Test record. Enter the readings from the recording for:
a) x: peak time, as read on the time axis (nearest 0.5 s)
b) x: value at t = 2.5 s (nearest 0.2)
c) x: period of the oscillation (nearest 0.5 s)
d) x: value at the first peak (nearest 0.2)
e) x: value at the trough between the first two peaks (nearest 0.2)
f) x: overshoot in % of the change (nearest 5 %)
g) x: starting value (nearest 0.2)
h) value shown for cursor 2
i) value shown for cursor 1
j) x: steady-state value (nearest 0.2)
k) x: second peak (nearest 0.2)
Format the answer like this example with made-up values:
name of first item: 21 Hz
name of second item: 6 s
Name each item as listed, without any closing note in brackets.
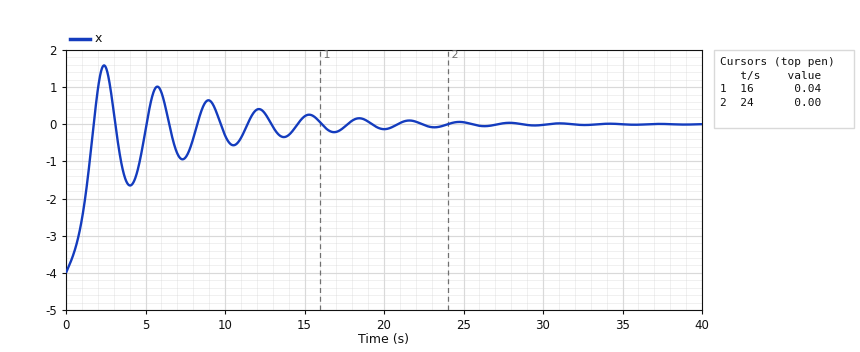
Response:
x: peak time, as read on the time axis: 2.5 s
x: value at t = 2.5 s: 1.6
x: period of the oscillation: 3.5 s
x: value at the first peak: 1.6
x: value at the trough between the first two peaks: -1.6
x: overshoot in % of the change: 40 %
x: starting value: -4.0
value shown for cursor 2: 0.00
value shown for cursor 1: 0.04
x: steady-state value: 0.0
x: second peak: 1.0
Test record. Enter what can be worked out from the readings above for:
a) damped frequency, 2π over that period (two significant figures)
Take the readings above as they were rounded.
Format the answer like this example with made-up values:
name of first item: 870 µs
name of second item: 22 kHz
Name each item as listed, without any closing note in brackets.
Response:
damped frequency, 2π over that period: 1.8 rad/s
